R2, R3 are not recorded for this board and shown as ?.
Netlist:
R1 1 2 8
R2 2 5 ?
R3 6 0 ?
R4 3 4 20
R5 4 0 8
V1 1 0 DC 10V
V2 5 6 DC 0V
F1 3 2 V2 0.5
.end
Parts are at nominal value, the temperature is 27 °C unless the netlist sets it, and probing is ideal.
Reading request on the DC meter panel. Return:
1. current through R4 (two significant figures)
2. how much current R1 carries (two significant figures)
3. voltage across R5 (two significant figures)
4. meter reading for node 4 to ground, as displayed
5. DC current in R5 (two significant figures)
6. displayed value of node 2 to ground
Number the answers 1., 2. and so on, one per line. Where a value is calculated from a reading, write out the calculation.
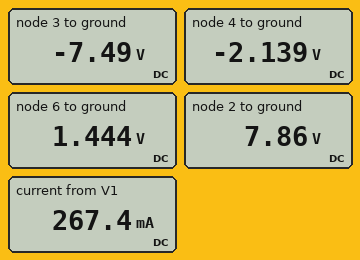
1. (-2.139 V - (-7.49 V)) / 20 Ω = 270 mA
2. (10 V - 7.86 V) / 8 Ω = 270 mA
3. 0 V - (-2.139 V) = 2.1 V
4. -2.139 V
5. (0 V - (-2.139 V)) / 8 Ω = 270 mA
6. 7.86 V
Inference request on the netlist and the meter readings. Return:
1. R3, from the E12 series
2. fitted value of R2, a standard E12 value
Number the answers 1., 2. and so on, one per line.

1. 2.7 Ω
2. 12 Ω
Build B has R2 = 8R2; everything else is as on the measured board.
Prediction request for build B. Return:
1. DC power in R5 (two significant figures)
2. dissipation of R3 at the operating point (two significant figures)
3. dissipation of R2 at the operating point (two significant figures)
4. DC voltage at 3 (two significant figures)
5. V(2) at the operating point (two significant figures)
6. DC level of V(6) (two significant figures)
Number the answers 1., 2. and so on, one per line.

1. 900 mW
2. 1.2 W
3. 3.7 W
4. -9.4 V
5. 7.3 V
6. 1.8 V
